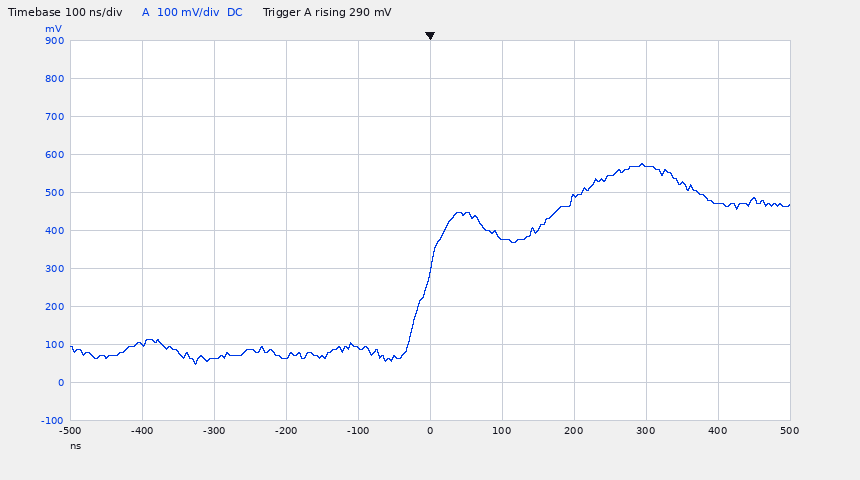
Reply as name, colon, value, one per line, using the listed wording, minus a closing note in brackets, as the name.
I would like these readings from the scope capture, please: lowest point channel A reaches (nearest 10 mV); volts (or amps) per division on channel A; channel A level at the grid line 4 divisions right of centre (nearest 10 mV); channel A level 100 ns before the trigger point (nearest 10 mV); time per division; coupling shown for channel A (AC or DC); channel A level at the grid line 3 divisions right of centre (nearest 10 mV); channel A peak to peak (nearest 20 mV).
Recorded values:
lowest point channel A reaches: 50 mV
volts (or amps) per division on channel A: 100 mV
channel A level at the grid line 4 divisions right of centre: 470 mV
channel A level 100 ns before the trigger point: 90 mV
time per division: 100 ns
coupling shown for channel A: DC
channel A level at the grid line 3 divisions right of centre: 570 mV
channel A peak to peak: 520 mV
